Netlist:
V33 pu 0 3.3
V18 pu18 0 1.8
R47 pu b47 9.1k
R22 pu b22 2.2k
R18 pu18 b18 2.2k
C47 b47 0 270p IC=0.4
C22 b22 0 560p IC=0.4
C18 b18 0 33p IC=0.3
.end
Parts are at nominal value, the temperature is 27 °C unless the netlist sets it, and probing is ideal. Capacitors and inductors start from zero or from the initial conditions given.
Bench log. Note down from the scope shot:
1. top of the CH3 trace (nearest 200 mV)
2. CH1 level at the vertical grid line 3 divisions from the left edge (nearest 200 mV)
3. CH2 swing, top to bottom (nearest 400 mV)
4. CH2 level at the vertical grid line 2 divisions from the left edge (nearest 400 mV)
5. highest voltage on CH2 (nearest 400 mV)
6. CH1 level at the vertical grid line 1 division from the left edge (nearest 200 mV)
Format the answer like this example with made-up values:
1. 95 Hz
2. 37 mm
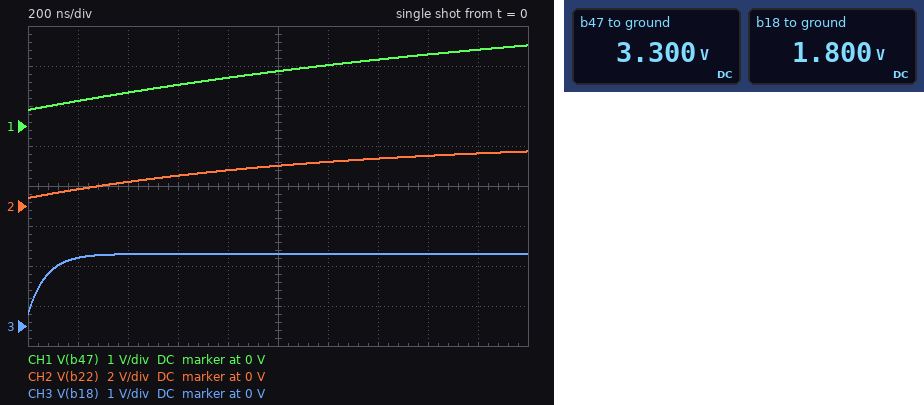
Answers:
1. 1.8 V
2. 1.0 V
3. 2.4 V
4. 1.2 V
5. 2.8 V
6. 600 mV
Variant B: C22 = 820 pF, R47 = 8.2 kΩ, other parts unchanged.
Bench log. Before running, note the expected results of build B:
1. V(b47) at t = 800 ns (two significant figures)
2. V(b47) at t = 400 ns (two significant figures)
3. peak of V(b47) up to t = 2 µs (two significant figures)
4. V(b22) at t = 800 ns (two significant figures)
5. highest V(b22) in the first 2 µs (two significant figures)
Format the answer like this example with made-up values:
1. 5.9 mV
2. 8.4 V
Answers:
1. 1.3 V
2. 880 mV
3. 2.1 V
4. 1.4 V
5. 2.3 V
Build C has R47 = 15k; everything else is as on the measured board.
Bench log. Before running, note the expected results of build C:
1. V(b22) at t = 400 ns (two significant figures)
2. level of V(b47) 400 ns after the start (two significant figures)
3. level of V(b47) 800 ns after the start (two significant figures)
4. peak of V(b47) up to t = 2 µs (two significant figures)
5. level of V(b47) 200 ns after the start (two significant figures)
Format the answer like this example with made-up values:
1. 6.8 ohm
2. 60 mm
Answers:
1. 1.2 V
2. 670 mV
3. 920 mV
4. 1.5 V
5. 540 mV
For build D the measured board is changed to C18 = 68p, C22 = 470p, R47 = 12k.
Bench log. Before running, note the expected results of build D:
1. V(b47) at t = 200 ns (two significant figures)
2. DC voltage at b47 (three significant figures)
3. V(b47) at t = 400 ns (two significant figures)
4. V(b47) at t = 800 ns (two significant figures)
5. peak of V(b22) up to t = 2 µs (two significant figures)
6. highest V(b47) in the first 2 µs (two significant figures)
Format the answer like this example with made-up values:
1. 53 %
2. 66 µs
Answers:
1. 570 mV
2. 3.30 V
3. 740 mV
4. 1.0 V
5. 2.9 V
6. 1.7 V
